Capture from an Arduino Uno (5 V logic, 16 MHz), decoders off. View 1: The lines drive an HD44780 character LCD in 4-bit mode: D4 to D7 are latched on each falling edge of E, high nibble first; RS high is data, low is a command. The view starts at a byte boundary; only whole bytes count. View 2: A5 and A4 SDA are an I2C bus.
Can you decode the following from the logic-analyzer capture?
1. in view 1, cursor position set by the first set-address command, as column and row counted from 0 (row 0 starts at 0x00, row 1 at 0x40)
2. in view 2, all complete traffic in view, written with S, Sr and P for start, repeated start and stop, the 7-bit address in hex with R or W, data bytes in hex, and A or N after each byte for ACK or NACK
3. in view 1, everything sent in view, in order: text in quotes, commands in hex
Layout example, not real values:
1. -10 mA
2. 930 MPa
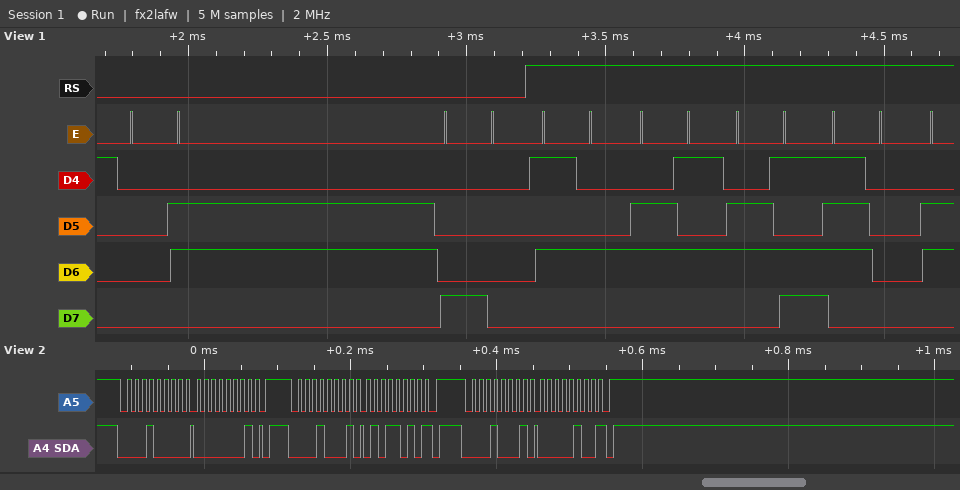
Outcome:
1. column 0, row 0
2. S 08W A 01 A P S 08R A 5A N P S 08R A 04 N P
3. 0x06 0x80 "Temp"
